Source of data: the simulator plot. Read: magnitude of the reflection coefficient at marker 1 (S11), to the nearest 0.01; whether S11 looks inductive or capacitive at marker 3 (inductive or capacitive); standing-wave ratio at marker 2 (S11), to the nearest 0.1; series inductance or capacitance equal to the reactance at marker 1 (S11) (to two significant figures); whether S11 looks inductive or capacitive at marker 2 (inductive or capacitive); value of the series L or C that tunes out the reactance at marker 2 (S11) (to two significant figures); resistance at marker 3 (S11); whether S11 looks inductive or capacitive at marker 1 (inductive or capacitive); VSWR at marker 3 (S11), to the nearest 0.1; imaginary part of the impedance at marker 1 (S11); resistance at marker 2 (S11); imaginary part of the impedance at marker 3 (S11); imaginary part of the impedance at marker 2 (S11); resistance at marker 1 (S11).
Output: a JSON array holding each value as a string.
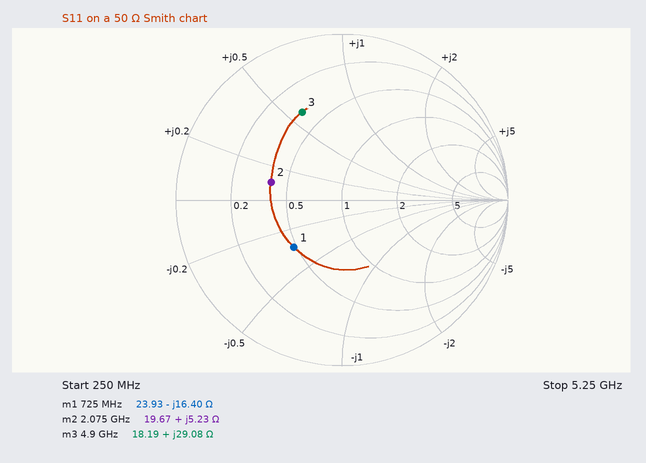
["0.41", "inductive", "2.6", "13 pF", "inductive", "15 pF", "18.19 Ω", "capacitive", "3.8", "-16.40 Ω", "19.67 Ω", "+29.08 Ω", "+5.23 Ω", "23.93 Ω"]
